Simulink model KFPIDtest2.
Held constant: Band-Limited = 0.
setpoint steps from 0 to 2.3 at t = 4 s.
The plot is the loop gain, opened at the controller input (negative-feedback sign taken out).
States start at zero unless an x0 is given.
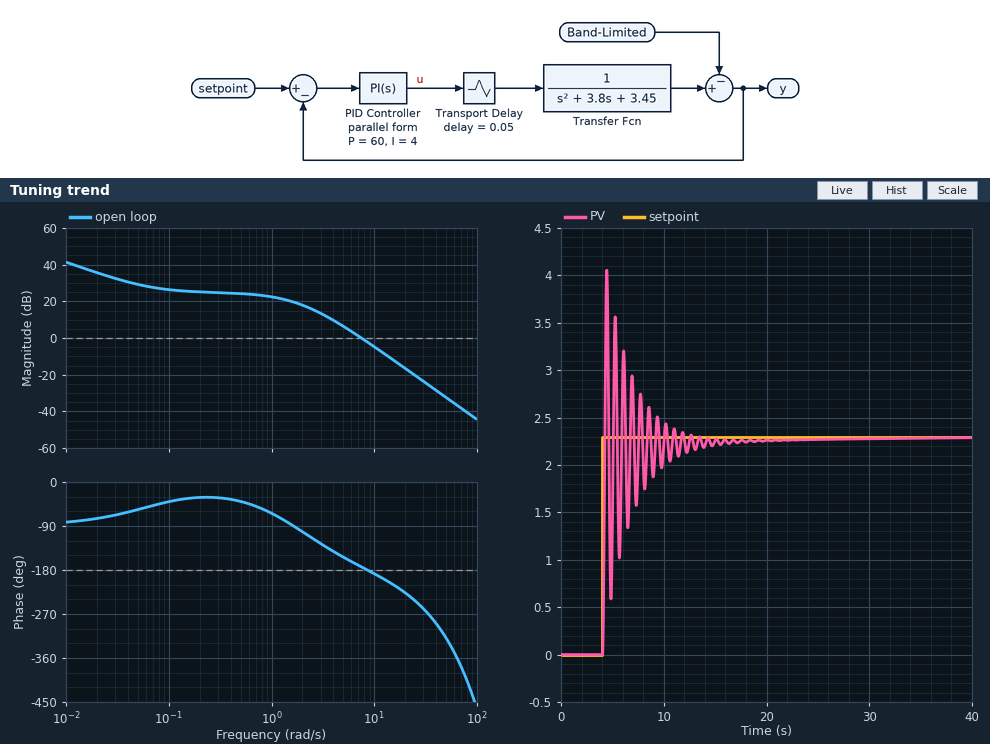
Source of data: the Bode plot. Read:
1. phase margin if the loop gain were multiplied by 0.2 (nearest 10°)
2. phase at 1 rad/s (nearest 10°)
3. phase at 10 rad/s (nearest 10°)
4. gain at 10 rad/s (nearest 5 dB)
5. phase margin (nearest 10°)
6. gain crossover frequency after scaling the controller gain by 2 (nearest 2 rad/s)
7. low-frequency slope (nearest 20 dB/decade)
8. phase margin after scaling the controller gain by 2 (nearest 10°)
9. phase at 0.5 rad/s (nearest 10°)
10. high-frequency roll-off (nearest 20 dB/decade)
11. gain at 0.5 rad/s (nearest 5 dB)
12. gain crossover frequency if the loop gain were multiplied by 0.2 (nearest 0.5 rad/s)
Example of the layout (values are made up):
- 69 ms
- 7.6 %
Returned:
- 60°
- -60°
- -190°
- -5 dB
- 10°
- 10 rad/s
- -20 dB/decade
- -10°
- -40°
- -40 dB/decade
- 25 dB
- 3.0 rad/s
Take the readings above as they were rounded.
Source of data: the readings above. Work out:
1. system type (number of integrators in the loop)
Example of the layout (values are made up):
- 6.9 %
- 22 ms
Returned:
- 1
